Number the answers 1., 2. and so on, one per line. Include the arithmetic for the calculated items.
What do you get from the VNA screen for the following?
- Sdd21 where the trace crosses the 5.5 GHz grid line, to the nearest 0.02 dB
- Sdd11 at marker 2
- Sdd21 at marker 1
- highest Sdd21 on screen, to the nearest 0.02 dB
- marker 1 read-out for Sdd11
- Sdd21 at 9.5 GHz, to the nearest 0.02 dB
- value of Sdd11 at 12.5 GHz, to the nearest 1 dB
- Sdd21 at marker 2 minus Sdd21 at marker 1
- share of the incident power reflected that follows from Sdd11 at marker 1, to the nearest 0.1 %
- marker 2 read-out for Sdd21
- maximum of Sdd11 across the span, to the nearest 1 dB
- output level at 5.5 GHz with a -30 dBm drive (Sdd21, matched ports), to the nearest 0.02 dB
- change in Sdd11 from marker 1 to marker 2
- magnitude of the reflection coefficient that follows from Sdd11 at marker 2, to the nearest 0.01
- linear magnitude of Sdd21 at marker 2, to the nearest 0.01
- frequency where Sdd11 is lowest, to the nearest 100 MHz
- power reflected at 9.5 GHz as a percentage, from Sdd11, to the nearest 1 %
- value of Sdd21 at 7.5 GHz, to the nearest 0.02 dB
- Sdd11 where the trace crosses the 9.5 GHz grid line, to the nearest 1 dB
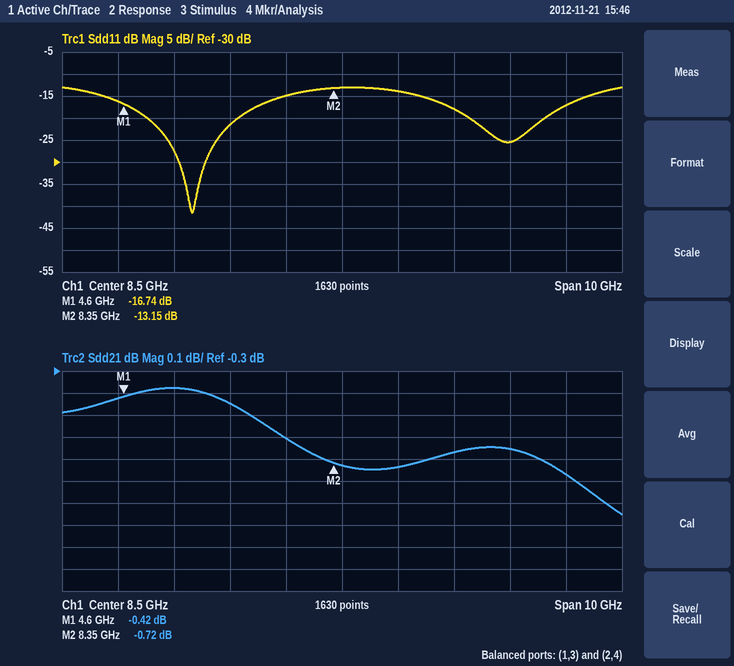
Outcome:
1. -0.38 dB
2. -13.15 dB
3. -0.42 dB
4. -0.38 dB
5. -16.74 dB
6. -0.74 dB
7. -17 dB
8. -0.72 − (-0.42) = -0.30 dB
9. 10^(-16.74/10) ≈ 2.1 %
10. -0.72 dB
11. -13 dB
12. -30 dBm + (-0.38 dB) = -30.38 dBm
13. -13.15 − (-16.74) = 3.59 dB
14. 10^(-13.15/20) ≈ 0.22
15. 10^(-0.72/20) ≈ 0.92
16. 5.8 GHz
17. 10^(-14/10) ≈ 4 %
18. -0.60 dB
19. -14 dB
